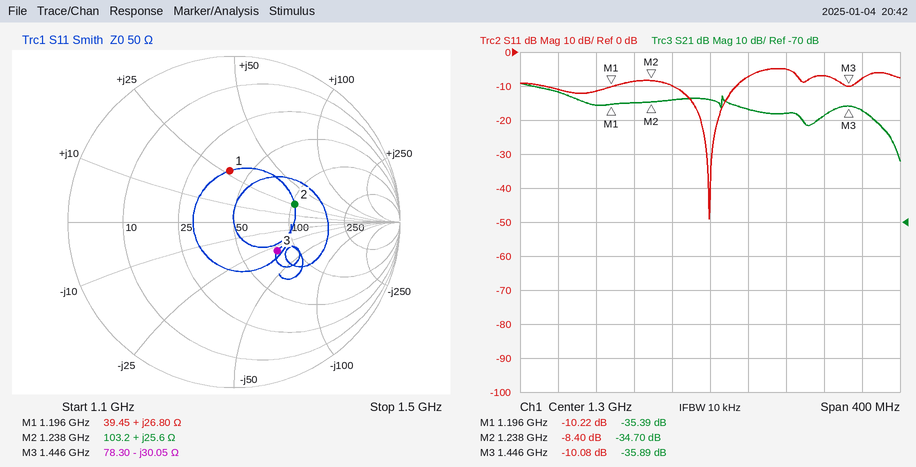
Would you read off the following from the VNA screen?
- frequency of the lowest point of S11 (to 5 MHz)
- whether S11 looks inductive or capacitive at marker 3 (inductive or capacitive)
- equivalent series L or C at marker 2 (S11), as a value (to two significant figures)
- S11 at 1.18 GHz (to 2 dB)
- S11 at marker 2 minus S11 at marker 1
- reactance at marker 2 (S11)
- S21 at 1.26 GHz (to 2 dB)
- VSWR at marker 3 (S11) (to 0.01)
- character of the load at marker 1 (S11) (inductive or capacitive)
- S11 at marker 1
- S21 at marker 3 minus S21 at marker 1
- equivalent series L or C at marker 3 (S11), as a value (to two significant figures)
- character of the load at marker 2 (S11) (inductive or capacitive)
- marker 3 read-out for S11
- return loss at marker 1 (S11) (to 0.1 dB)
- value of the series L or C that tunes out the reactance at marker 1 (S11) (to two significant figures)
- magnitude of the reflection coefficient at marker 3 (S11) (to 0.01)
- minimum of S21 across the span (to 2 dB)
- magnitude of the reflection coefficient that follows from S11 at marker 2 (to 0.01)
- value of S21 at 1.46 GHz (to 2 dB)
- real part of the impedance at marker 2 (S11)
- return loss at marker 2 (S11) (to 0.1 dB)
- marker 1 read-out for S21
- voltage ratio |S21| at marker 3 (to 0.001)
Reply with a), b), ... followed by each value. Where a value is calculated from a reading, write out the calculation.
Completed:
a) 1.300 GHz
b) capacitive
c) L = 25.6 Ω/(2π × 1.238 GHz) ≈ 3.3 nH
d) -12 dB
e) -8.4 − (-10.22) = 1.82 dB
f) +25.6 Ω
g) -34 dB
h) 1.91
i) inductive
j) -10.22 dB
k) -35.89 − (-35.39) = -0.50 dB
l) C = 1/(2π × 1.446 GHz × 30.05 Ω) ≈ 3.7 pF
m) inductive
n) -10.08 dB
o) 10.2 dB
p) C = 1/(2π × 1.196 GHz × 26.8 Ω) ≈ 5.0 pF
q) 10^(-10.08/20) ≈ 0.31
r) -52 dB
s) 10^(-8.4/20) ≈ 0.38
t) -38 dB
u) 103.2 Ω
v) 8.4 dB
w) -35.39 dB
x) 10^(-35.89/20) ≈ 0.016
